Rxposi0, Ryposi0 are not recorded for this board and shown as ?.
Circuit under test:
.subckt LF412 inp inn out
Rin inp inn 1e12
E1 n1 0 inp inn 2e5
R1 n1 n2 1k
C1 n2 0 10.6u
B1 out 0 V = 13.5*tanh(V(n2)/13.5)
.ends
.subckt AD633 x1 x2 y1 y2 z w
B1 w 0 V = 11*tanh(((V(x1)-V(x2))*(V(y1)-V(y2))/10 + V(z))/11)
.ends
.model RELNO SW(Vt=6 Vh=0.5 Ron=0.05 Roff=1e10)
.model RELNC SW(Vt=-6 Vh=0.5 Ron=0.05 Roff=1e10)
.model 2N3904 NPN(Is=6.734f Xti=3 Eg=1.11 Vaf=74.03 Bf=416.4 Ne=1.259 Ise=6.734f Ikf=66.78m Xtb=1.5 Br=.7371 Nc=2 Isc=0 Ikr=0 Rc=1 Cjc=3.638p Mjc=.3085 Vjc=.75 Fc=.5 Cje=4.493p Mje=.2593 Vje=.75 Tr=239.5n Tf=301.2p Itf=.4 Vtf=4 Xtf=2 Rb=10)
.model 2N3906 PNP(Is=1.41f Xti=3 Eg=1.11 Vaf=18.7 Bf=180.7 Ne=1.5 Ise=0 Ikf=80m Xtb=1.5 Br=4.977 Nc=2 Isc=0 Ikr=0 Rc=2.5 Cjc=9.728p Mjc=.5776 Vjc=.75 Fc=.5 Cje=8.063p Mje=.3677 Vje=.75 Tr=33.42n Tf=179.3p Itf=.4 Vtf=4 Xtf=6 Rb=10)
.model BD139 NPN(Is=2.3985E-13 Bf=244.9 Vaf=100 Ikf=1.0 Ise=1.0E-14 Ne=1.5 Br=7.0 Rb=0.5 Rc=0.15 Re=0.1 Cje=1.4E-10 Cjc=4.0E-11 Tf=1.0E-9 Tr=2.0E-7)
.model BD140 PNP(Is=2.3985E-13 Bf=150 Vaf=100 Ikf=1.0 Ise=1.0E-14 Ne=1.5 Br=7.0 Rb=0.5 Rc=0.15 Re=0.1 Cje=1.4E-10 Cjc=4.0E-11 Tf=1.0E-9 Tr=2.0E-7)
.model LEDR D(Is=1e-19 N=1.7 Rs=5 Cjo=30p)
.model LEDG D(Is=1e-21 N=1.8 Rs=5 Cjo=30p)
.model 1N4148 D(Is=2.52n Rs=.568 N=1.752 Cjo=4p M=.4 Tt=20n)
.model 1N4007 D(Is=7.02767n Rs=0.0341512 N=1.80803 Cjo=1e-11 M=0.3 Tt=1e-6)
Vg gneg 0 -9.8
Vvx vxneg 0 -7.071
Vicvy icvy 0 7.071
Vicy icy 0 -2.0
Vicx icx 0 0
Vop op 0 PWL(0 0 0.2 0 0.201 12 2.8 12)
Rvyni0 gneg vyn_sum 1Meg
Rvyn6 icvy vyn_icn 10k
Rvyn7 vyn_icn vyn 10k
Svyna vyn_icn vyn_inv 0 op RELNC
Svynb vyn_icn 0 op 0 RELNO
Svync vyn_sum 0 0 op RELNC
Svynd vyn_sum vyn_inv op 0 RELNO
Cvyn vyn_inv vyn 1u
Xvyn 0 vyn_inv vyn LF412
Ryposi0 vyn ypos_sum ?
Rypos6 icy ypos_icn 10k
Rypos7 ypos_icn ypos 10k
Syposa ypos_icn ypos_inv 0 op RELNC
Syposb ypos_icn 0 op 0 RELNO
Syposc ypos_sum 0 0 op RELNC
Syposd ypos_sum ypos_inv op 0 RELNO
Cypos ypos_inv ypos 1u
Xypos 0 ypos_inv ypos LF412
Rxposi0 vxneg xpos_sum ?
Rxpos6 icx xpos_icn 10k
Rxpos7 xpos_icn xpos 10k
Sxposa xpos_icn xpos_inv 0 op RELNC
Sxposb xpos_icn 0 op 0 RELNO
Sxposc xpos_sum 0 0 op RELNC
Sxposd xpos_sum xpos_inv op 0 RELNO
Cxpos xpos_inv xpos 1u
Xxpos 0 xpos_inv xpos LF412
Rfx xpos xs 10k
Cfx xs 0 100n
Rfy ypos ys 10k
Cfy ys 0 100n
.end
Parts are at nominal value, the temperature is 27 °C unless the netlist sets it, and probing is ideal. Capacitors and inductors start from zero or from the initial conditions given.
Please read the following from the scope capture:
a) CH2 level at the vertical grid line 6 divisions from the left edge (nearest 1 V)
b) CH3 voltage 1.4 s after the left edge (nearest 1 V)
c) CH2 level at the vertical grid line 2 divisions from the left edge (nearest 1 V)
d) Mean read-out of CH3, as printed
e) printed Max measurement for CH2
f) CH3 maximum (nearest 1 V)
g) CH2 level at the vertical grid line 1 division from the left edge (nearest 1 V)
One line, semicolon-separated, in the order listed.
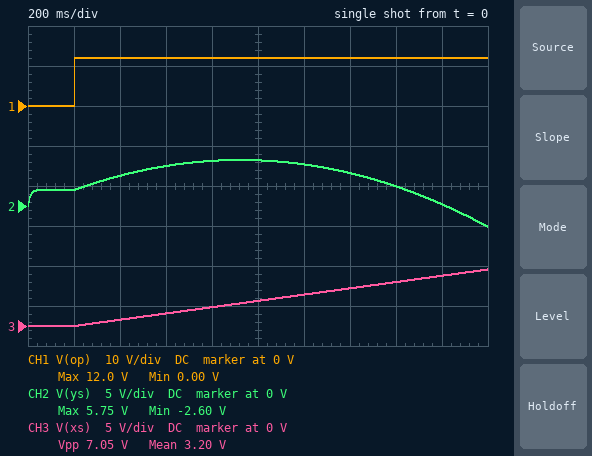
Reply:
5 V; 5 V; 4 V; 3.20 V; 5.75 V; 7 V; 2 V
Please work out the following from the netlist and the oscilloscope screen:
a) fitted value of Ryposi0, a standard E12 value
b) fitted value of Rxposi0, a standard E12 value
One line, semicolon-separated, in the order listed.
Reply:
680 kΩ; 1.8 MΩ
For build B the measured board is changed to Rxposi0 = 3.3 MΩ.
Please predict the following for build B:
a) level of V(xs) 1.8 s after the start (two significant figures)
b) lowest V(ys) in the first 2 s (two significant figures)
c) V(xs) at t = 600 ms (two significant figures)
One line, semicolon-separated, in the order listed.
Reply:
3.4 V; -2.6 V; 850 mV
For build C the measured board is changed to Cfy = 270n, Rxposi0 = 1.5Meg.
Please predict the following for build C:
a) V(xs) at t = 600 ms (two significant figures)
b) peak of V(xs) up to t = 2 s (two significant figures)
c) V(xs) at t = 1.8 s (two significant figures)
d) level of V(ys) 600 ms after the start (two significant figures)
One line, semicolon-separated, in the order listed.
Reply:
1.9 V; 8.5 V; 7.5 V; 5.0 V
